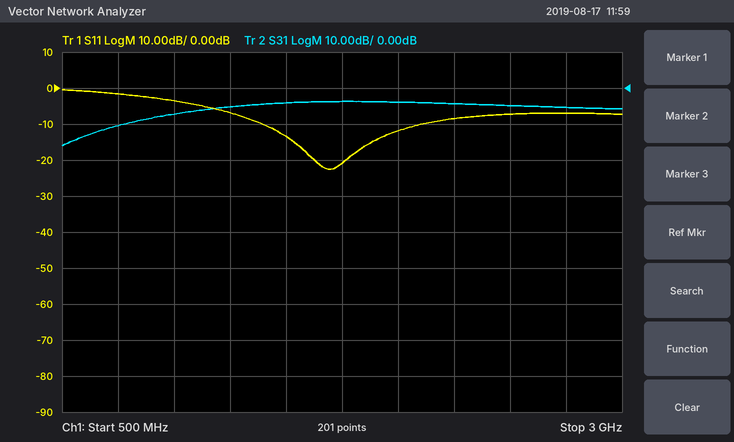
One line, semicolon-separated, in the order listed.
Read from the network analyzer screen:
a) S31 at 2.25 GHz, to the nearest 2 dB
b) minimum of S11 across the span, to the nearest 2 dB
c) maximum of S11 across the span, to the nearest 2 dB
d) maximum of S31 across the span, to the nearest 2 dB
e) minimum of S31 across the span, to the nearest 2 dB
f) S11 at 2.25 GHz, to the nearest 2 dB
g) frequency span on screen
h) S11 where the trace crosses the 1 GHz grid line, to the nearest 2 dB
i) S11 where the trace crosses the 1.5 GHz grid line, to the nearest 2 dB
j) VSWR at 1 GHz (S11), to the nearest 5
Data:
-4 dB; -22 dB; 0 dB; -4 dB; -16 dB; -8 dB; 2.5 GHz; -4 dB; -14 dB; 5
